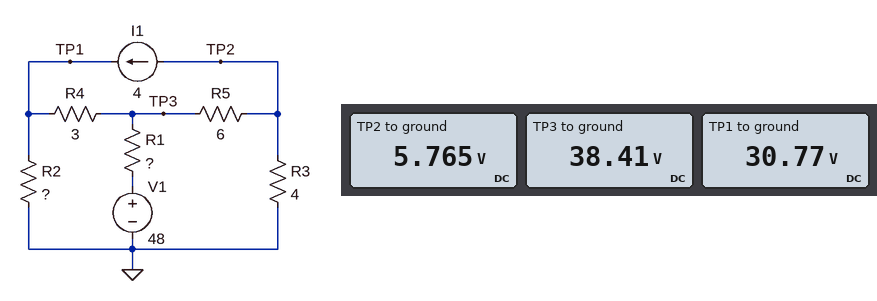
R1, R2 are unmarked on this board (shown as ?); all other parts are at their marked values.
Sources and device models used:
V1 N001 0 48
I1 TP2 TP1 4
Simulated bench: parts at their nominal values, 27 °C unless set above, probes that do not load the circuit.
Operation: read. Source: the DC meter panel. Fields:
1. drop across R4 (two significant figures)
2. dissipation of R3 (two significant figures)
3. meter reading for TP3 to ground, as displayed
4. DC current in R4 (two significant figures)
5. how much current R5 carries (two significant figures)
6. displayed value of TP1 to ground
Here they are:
7.6 V
8.3 W
38.41 V
2.5 A
5.4 A
30.77 V
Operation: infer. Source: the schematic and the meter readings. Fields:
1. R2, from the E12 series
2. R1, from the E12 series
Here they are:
4.7 Ω
1.2 Ω
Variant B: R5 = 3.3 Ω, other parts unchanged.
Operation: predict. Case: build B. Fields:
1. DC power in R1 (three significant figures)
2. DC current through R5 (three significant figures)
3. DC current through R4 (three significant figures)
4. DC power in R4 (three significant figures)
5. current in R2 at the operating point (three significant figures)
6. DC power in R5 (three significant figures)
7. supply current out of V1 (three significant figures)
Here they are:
109 W
7.20 A
2.31 A
16.0 W
6.31 A
171 W
9.51 A
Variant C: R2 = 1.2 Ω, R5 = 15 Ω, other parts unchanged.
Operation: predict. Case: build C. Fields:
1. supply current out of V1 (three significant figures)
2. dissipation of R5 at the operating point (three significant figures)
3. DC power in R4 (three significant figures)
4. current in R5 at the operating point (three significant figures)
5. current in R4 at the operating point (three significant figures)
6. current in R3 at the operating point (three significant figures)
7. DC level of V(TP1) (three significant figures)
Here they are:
10.1 A
112 W
164 W
2.73 A
7.39 A
1.27 A
13.7 V
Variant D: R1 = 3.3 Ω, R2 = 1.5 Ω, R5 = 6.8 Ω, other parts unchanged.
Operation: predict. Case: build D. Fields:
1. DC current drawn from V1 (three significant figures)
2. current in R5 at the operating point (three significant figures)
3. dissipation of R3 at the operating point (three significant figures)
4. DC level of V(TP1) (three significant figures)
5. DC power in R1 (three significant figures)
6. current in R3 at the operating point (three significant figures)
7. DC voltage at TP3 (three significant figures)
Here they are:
7.48 A
3.64 A
521 mW
11.8 V
185 W
361 mA
23.3 V
